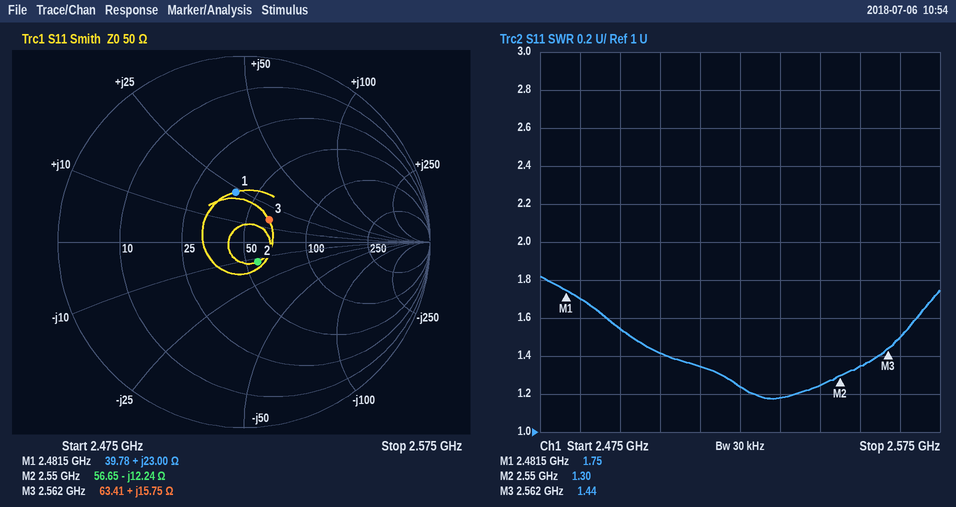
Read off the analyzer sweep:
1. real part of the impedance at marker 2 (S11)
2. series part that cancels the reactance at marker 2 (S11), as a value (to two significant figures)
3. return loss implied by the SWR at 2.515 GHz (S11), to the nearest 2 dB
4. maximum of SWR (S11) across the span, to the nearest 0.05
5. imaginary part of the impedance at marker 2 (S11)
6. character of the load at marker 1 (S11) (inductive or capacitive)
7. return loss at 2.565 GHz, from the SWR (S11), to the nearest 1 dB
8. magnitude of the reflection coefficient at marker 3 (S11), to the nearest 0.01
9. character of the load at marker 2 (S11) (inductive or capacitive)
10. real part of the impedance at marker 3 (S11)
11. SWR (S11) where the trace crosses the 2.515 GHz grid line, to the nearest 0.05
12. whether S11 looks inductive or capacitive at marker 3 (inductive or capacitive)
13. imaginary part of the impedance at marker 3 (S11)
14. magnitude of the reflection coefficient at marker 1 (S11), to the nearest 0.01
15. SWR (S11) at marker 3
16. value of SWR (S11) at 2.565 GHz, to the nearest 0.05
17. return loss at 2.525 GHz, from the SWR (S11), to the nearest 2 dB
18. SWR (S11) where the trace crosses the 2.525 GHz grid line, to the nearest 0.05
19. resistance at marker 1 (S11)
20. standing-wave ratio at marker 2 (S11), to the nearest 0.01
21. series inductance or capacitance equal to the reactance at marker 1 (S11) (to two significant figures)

56.65 Ω
760 pH
16 dB
1.80
-12.24 Ω
inductive
14 dB
0.18
capacitive
63.41 Ω
1.35
inductive
+15.75 Ω
0.27
1.44
1.50
20 dB
1.25
39.78 Ω
1.30
1.5 nH
